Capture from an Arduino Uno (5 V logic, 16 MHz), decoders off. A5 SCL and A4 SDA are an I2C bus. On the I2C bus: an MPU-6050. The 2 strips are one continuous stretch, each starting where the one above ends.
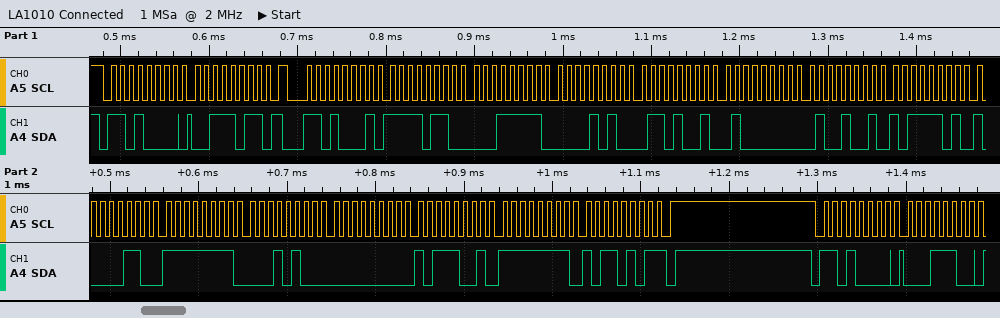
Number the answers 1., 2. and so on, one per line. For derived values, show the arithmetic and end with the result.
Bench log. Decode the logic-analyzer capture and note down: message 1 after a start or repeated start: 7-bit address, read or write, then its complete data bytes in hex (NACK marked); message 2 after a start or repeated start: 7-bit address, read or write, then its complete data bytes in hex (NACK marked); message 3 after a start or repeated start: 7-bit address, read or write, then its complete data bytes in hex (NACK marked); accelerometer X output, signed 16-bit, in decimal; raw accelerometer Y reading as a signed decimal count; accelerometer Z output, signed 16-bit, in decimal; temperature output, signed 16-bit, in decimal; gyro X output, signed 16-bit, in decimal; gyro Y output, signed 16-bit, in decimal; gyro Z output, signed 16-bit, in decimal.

1. 0x68 write: 3B
2. 0x68 read: F6 1F 0A 69 40 49 BD 86 FF 14 00 B9 FF B5 NACK
3. 0x68 write: 1C
4. 0xF61F = -2529
5. 0x0A69 = 2665
6. 0x4049 = 16457
7. 0xBD86 = -17018
8. 0xFF14 = -236
9. 0x00B9 = 185
10. 0xFFB5 = -75
